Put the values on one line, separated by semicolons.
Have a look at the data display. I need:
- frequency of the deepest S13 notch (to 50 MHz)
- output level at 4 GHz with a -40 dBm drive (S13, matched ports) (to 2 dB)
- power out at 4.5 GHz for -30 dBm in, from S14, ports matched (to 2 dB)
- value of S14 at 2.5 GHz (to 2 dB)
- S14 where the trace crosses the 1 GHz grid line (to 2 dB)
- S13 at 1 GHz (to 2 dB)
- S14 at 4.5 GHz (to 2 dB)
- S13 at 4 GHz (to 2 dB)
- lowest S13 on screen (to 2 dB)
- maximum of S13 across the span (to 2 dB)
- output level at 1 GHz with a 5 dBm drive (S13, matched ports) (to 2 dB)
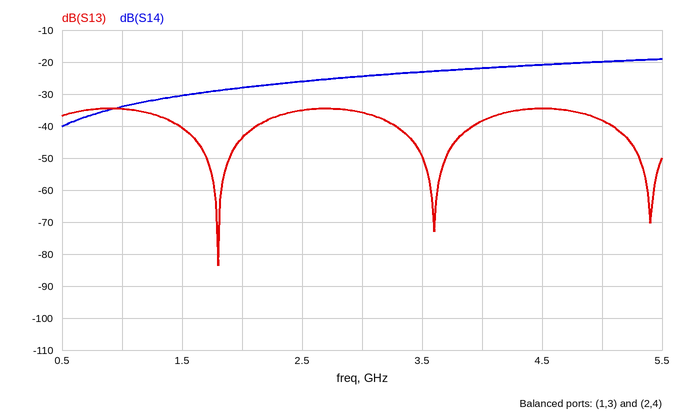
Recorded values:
1.80 GHz; -78 dBm; -50 dBm; -26 dB; -34 dB; -34 dB; -20 dB; -38 dB; -84 dB; -34 dB; -30 dBm
